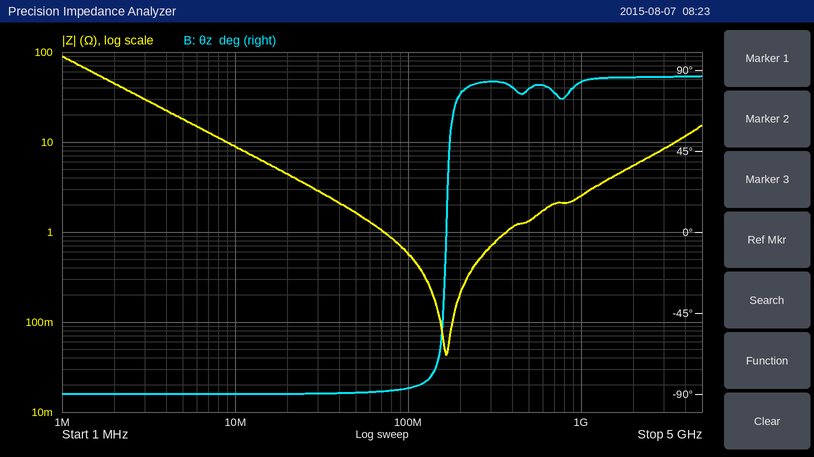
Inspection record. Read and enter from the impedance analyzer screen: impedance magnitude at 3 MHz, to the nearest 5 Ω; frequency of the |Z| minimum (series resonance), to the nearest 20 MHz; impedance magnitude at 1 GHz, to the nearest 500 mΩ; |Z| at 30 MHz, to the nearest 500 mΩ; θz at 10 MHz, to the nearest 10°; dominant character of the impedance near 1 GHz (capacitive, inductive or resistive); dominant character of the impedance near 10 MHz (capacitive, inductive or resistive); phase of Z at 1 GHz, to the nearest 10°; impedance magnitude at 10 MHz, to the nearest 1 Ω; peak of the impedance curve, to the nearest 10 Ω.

30 Ω
160 MHz
2.5 Ω
3.0 Ω
-90°
inductive
capacitive
80°
9 Ω
90 Ω
